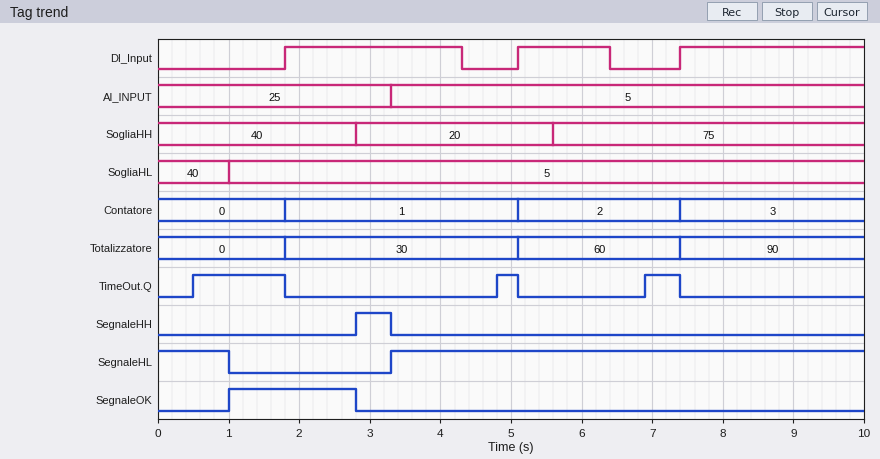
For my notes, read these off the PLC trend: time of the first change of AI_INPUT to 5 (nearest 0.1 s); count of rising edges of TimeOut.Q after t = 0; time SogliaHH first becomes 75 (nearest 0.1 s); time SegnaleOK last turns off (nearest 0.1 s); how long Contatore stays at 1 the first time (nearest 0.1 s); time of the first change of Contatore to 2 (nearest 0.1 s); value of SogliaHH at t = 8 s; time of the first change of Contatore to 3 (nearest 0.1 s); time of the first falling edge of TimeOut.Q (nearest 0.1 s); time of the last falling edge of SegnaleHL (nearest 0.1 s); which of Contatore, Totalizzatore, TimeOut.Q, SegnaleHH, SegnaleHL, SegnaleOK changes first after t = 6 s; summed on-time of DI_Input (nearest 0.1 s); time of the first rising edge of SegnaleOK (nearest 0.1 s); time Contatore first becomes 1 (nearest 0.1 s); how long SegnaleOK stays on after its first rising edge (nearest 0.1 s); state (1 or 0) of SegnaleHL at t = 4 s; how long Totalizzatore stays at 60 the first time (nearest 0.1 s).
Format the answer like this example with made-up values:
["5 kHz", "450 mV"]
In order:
["3.3 s", "3", "5.6 s", "2.8 s", "3.3 s", "5.1 s", "75", "7.4 s", "1.8 s", "1.0 s", "TimeOut.Q", "6.4 s", "1.0 s", "1.8 s", "1.8 s", "1", "2.3 s"]
